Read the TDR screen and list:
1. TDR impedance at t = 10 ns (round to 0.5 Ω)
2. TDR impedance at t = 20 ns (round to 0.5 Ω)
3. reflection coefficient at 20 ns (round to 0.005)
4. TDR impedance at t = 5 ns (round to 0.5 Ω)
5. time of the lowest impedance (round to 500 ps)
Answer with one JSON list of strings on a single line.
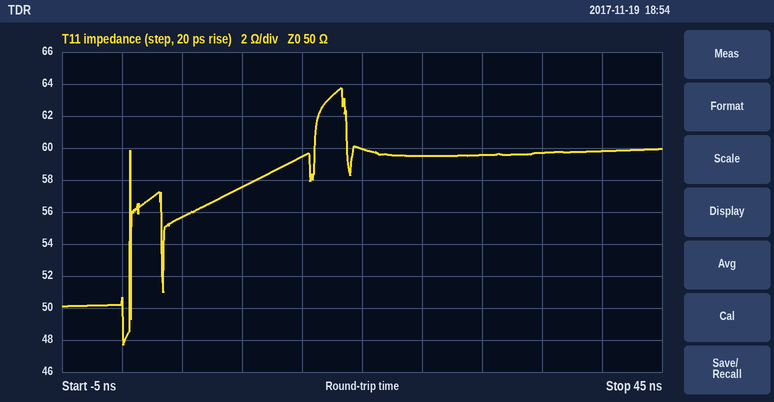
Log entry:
["57.5 Ω", "60.0 Ω", "+0.090", "55.5 Ω", "0.0 ns"]
